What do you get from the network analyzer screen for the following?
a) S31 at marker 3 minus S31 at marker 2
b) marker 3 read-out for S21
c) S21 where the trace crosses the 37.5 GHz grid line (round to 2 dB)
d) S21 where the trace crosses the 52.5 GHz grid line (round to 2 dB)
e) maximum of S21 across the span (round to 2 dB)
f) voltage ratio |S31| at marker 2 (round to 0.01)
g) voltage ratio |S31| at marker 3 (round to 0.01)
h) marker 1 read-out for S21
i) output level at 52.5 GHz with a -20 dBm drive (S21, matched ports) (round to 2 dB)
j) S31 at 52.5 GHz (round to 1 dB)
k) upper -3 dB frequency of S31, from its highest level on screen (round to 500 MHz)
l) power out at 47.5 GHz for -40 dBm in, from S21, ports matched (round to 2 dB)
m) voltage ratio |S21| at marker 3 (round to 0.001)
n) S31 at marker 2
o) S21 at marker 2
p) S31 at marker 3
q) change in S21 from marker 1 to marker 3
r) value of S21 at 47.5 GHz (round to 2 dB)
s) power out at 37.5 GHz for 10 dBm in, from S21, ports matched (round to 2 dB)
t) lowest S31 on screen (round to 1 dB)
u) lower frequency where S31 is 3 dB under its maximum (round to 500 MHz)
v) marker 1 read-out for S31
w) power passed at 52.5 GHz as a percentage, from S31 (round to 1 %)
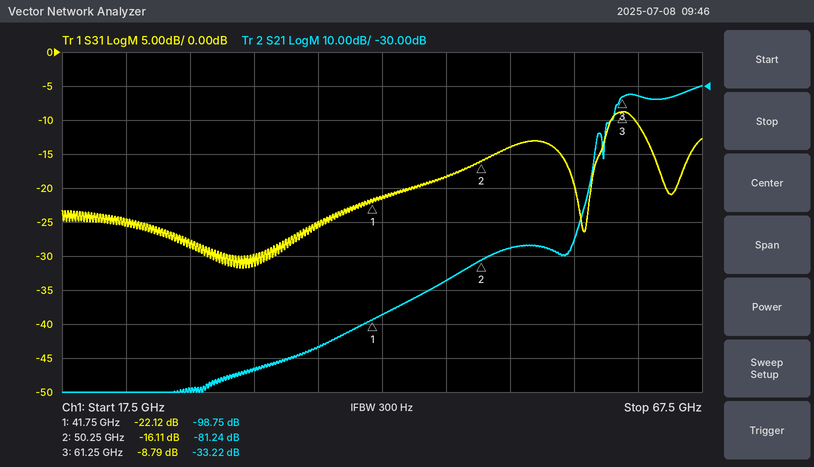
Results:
7.32 dB
-33.22 dB
-106 dB
-78 dB
-30 dB
0.16
0.36
-98.75 dB
-98 dBm
-14 dB
63.0 GHz
-128 dBm
0.022
-16.11 dB
-81.24 dB
-8.79 dB
65.53 dB
-88 dB
-96 dBm
-32 dB
60.0 GHz
-22.12 dB
4 %
